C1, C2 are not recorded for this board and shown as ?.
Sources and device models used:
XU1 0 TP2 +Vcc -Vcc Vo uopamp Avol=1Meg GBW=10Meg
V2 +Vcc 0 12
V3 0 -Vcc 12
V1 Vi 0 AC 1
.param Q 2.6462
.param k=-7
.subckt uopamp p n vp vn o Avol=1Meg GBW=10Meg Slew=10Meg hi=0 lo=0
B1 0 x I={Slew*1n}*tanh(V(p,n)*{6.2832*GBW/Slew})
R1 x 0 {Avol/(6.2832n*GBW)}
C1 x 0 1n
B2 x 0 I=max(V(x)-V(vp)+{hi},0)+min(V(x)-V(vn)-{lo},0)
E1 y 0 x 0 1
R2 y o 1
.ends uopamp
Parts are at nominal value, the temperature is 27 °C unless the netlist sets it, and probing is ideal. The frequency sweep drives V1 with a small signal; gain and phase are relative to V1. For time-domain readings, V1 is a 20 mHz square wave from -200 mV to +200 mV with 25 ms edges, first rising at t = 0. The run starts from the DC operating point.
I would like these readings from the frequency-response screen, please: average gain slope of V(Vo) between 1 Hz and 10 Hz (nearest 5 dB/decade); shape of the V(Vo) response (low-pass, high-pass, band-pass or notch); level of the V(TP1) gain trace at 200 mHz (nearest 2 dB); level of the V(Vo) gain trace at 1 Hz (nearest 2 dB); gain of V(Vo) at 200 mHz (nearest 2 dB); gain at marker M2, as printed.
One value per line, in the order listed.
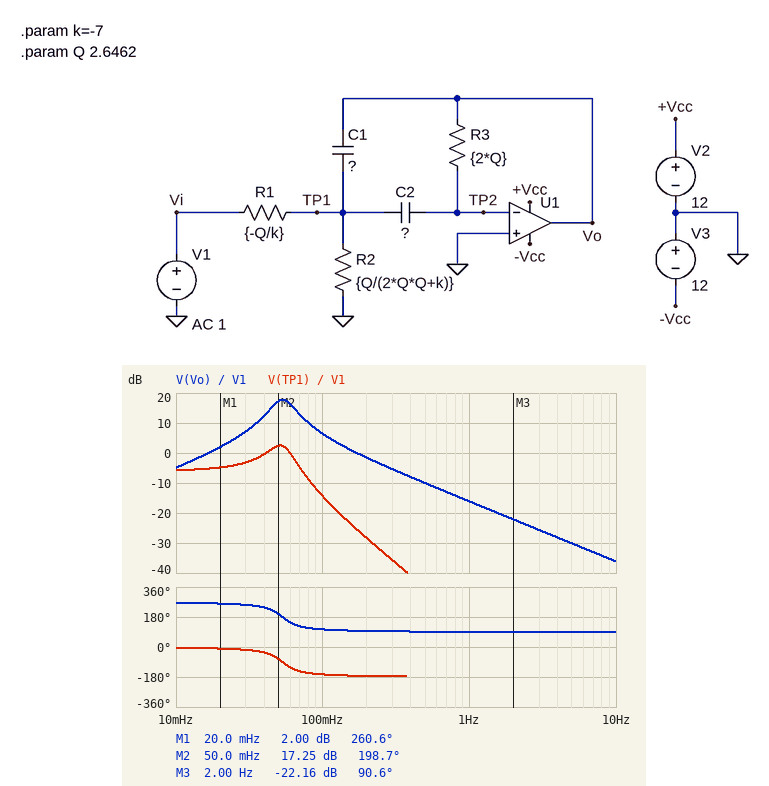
-20 dB/decade
band-pass
-28 dB
-16 dB
-2 dB
17.25 dB
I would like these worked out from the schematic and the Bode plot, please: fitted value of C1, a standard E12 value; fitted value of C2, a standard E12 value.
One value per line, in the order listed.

2.7 F
3.3 F
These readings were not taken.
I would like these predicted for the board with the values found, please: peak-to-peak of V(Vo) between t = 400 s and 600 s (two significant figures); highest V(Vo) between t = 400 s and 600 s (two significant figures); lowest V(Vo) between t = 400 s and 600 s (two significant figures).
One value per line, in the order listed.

1.8 V
910 mV
-910 mV
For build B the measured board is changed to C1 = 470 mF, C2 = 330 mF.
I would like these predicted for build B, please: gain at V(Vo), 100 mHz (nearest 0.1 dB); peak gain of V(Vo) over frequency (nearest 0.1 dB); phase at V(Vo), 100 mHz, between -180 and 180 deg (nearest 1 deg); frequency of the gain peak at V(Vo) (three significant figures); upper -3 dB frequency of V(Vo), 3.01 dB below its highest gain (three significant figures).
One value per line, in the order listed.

-4.7 dB
15.2 dB
-96 deg
404 mHz
489 mHz
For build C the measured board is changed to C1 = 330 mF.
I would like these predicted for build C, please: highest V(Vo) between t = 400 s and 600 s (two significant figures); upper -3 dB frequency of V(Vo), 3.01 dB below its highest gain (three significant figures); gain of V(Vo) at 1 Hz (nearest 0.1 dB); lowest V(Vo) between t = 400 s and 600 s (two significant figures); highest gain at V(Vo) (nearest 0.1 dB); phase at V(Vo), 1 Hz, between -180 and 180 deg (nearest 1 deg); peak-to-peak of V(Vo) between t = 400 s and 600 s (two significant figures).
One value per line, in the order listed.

2.2 V
211 mHz
2.3 dB
-2.2 V
22.1 dB
96 deg
4.4 V
